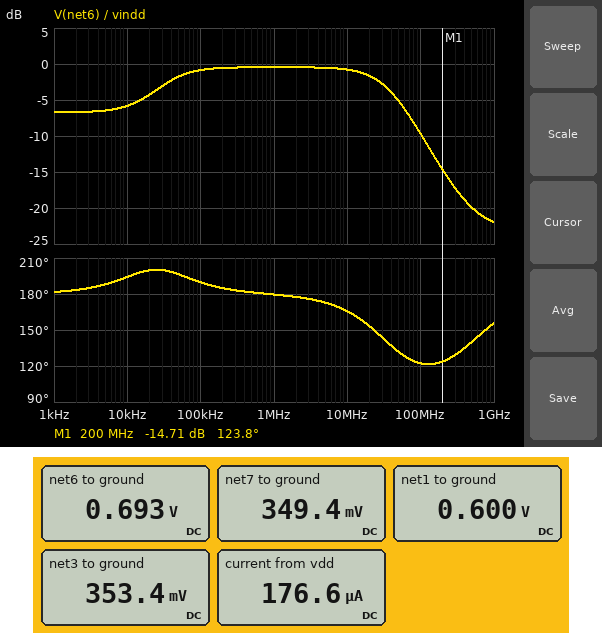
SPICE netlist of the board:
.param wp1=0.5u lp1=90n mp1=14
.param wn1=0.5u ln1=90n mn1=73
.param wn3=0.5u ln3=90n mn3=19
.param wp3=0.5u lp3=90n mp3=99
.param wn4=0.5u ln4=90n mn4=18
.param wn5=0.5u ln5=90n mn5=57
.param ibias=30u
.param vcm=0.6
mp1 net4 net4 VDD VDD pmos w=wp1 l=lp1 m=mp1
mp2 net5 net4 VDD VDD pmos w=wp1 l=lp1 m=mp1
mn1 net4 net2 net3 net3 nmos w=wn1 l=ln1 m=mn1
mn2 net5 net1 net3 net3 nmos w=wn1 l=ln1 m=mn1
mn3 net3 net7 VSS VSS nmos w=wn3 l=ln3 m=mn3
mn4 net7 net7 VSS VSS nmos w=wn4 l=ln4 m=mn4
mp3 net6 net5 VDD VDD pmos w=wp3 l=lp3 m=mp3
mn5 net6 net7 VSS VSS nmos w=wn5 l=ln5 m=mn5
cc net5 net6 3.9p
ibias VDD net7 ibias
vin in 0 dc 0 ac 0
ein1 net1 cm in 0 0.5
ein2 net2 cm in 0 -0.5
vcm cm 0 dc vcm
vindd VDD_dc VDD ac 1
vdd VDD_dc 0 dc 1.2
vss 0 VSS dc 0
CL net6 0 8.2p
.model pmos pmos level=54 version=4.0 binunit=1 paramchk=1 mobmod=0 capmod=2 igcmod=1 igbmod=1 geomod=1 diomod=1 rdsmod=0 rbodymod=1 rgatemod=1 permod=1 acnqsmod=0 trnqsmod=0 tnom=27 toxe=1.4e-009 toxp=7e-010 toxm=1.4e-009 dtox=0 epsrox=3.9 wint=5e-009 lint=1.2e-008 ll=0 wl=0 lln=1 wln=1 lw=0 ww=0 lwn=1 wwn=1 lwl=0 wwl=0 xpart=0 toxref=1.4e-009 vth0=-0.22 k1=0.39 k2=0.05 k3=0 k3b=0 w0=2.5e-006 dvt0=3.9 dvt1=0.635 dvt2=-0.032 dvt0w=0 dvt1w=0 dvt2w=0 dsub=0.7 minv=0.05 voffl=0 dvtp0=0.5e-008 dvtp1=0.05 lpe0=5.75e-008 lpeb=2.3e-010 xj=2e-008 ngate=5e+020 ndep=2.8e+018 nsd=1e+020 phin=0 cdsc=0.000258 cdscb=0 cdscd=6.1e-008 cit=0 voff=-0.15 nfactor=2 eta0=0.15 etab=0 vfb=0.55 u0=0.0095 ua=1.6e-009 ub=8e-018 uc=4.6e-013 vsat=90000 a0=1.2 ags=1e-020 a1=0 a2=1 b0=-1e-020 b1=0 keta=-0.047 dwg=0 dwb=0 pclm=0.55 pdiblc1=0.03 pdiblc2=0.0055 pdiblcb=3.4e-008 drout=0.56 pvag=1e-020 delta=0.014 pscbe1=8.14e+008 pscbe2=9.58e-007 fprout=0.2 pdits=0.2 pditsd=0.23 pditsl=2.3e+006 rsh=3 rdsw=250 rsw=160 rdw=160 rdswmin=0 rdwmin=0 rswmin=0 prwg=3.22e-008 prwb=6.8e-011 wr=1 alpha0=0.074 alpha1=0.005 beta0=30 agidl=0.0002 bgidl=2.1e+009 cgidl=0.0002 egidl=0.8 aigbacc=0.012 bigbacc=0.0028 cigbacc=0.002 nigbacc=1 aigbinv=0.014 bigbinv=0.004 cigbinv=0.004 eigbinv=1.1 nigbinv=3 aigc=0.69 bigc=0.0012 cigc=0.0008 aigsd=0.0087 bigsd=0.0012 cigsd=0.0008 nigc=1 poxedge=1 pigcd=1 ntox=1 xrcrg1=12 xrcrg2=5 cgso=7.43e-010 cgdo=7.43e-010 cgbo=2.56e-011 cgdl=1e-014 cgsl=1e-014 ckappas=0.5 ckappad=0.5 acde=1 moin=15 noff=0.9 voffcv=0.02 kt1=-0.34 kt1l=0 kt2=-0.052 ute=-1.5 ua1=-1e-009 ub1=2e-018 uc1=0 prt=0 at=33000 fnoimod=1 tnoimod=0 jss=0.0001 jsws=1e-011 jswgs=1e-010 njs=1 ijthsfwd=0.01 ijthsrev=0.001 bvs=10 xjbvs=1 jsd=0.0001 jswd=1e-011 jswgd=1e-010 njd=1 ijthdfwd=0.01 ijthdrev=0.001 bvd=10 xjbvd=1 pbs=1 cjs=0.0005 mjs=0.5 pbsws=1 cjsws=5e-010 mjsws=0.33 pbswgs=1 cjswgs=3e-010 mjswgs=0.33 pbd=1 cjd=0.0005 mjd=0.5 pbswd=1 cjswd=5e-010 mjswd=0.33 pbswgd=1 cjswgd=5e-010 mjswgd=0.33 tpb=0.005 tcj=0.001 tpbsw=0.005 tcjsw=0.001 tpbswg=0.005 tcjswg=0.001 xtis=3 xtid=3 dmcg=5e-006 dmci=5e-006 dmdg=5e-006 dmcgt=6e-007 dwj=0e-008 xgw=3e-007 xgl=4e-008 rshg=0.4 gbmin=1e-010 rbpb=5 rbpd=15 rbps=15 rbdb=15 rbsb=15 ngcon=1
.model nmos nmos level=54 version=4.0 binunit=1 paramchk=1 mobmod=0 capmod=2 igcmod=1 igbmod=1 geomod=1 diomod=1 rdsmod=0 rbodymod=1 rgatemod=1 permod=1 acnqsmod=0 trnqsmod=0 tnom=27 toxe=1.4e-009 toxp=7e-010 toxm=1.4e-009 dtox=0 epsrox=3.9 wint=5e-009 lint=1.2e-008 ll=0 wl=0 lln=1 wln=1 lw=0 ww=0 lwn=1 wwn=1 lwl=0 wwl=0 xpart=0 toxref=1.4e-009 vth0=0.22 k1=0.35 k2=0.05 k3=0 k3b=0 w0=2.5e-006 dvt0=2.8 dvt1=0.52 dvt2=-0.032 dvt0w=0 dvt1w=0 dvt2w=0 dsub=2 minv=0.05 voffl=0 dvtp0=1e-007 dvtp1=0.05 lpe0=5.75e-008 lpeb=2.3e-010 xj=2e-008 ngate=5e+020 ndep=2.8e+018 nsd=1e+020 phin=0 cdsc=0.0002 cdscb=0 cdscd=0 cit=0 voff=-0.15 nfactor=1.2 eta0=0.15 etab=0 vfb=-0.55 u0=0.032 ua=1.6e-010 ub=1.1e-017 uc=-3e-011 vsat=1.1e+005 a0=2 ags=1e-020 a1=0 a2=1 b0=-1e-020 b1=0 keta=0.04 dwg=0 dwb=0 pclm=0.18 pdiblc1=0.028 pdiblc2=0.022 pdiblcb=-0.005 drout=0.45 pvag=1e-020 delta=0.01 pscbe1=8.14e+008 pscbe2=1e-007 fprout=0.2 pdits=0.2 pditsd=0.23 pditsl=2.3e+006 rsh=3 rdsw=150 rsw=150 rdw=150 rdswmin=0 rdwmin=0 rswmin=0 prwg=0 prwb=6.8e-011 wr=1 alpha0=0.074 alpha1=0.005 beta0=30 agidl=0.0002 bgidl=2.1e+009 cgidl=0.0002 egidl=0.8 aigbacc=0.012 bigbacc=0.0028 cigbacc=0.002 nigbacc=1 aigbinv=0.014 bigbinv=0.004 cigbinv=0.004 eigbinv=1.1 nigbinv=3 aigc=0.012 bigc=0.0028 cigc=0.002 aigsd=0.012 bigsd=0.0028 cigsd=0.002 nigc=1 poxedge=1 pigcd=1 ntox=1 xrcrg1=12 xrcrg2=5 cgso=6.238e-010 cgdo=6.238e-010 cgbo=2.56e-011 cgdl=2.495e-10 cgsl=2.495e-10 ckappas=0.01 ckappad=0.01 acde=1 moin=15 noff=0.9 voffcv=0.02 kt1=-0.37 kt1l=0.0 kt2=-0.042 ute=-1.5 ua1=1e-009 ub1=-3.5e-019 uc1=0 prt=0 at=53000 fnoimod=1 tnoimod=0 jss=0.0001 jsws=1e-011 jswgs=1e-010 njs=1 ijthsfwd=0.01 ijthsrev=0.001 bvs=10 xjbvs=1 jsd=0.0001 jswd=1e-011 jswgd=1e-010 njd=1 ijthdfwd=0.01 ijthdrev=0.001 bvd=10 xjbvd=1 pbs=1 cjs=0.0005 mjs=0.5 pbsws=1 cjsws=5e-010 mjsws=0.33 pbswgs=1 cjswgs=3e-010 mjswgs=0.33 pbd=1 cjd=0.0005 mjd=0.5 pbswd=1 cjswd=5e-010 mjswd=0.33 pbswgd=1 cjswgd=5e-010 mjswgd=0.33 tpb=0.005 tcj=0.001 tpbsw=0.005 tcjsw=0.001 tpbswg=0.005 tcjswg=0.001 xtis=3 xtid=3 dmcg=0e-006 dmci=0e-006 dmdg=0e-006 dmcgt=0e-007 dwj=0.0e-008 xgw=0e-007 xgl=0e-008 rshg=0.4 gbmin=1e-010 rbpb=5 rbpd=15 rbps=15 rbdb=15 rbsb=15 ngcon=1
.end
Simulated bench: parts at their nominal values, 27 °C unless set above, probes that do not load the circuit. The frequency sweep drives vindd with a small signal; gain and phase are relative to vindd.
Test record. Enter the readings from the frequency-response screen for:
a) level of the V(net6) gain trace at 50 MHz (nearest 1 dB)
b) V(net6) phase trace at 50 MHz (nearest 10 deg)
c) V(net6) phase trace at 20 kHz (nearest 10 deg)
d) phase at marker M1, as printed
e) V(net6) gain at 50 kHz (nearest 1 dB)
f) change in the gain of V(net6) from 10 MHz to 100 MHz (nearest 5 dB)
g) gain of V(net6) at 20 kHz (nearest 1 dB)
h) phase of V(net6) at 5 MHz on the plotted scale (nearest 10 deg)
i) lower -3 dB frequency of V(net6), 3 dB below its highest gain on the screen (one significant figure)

-5 dB
130 deg
200 deg
123.8 deg
-2 dB
-10 dB
-4 dB
170 deg
30 kHz
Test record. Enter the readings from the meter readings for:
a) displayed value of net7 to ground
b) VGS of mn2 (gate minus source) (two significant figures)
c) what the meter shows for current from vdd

349.4 mV
250 mV
176.6 µA
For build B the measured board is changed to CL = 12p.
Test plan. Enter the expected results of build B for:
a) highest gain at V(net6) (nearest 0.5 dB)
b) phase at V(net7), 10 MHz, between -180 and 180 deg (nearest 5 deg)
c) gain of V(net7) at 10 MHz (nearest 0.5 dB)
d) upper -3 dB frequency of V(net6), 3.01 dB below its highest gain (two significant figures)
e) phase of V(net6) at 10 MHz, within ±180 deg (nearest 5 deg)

-0.5 dB
-145 deg
-51.5 dB
25 MHz
160 deg
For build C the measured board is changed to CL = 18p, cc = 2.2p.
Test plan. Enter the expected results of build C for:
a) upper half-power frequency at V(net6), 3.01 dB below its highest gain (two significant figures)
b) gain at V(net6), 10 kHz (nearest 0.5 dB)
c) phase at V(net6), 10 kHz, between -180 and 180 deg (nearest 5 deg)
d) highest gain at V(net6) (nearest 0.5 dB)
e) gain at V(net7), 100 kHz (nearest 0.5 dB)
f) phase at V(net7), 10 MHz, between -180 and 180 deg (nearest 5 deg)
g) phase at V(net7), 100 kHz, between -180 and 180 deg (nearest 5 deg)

17 MHz
-6.5 dB
-170 deg
-1.0 dB
-56.5 dB
-155 deg
-165 deg
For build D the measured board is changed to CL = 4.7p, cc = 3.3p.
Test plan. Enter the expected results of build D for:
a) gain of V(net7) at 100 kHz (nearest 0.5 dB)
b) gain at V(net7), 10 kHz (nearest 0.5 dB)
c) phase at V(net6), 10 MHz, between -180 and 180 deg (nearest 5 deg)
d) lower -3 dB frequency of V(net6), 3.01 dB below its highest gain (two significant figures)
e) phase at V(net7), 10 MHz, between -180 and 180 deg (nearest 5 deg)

-56.0 dB
-61.0 dB
170 deg
31 kHz
-135 deg
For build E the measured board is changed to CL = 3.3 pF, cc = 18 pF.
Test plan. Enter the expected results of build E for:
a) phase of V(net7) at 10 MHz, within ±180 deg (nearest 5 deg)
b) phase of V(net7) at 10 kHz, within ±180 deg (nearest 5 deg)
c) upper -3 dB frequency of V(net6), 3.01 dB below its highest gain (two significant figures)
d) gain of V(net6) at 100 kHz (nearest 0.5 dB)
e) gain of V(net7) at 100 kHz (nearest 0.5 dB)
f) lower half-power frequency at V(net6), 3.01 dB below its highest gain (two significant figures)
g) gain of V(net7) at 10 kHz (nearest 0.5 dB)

-135 deg
-160 deg
82 MHz
-0.5 dB
-55.0 dB
5.9 kHz
-56.5 dB
